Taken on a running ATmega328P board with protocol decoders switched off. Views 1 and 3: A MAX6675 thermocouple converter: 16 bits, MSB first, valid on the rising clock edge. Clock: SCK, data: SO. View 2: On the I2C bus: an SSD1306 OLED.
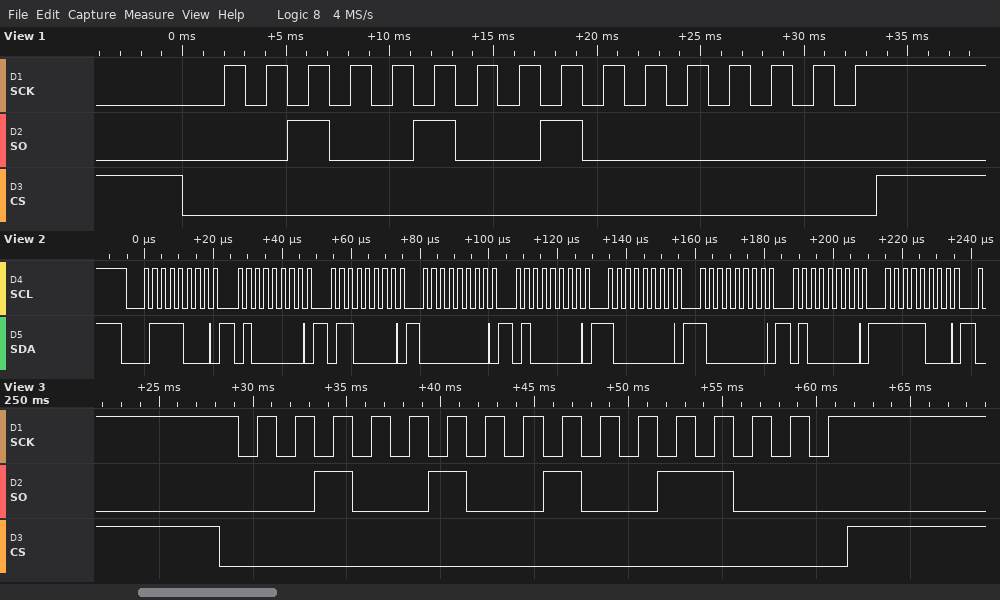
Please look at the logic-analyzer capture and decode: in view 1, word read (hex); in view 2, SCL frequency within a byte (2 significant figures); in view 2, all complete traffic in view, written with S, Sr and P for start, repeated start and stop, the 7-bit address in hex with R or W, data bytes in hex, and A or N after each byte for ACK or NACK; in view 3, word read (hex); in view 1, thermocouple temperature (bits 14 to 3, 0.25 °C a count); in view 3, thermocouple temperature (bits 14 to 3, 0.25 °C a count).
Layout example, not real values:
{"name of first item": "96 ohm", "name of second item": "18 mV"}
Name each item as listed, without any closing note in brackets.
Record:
{"in view 1, word read": "0x2480", "in view 2, SCL frequency within a byte": "400 kHz", "in view 2, all complete traffic in view, written with S, Sr and P for start, repeated start and stop, the 7-bit address in hex with R or W, data bytes in hex, and A or N after each byte for ACK or NACK": "S 3CW A 40 A 60 A 00 A 40 A 80 A 80 A 40 A F8 A", "in view 3, word read": "0x2498", "in view 1, thermocouple temperature": "292.00 °C", "in view 3, thermocouple temperature": "292.75 °C"}
